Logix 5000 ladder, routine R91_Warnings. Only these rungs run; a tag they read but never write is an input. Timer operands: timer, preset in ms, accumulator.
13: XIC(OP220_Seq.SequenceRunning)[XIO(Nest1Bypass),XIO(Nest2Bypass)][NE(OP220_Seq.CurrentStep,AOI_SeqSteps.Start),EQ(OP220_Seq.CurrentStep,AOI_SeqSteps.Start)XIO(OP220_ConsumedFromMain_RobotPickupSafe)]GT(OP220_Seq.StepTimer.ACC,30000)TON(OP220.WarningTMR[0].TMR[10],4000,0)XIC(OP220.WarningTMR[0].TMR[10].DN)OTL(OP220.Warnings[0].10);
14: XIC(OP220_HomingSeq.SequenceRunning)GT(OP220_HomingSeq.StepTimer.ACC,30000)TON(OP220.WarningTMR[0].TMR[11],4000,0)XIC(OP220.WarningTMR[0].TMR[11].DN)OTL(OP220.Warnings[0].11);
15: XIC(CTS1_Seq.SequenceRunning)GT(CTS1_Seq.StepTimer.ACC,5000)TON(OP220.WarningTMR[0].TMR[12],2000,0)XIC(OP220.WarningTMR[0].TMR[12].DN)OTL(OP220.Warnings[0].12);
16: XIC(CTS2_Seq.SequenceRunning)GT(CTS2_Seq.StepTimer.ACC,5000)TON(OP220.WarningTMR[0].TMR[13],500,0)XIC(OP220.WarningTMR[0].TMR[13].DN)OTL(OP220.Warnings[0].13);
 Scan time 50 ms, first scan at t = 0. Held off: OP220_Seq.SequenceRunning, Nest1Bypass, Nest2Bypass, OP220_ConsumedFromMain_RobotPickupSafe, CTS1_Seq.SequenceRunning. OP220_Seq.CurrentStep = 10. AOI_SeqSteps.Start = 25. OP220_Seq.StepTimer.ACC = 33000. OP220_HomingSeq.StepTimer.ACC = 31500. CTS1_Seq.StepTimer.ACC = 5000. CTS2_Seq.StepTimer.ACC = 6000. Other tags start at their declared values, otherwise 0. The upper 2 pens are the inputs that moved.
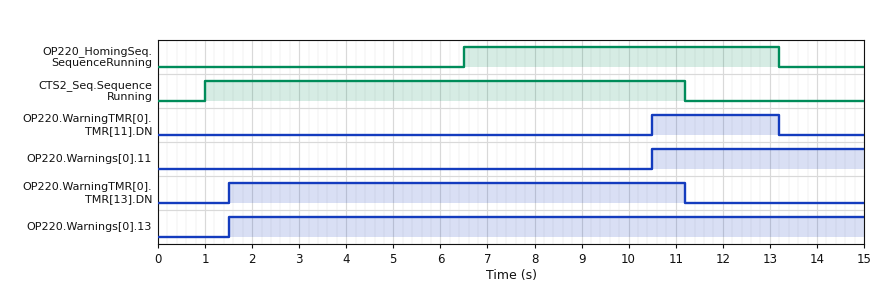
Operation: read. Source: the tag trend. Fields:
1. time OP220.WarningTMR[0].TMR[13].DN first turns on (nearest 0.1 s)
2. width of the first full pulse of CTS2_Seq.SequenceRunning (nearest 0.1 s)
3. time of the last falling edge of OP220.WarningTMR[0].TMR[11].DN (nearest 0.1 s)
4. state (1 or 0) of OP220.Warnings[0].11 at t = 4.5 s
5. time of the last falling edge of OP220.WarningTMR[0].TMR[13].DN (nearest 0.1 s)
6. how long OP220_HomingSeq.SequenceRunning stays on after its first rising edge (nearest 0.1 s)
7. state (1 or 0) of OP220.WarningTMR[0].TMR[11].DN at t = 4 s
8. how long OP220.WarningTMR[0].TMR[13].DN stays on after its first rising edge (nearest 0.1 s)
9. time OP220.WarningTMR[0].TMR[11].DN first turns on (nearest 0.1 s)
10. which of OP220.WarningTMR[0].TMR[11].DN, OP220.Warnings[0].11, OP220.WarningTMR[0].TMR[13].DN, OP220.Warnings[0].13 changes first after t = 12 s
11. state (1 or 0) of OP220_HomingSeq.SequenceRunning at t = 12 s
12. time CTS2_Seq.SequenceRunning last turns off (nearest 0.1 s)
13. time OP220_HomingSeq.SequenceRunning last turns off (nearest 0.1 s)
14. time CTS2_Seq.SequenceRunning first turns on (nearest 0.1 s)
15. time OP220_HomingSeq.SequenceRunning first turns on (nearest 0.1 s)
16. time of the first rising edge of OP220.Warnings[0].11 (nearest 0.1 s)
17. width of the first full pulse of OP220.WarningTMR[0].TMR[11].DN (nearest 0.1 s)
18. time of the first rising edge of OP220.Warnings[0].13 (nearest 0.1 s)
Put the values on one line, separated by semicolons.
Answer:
1.5 s; 10.2 s; 13.2 s; 0; 11.2 s; 6.7 s; 0; 9.7 s; 10.5 s; OP220.WarningTMR[0].TMR[11].DN; 1; 11.2 s; 13.2 s; 1.0 s; 6.5 s; 10.5 s; 2.7 s; 1.5 s
